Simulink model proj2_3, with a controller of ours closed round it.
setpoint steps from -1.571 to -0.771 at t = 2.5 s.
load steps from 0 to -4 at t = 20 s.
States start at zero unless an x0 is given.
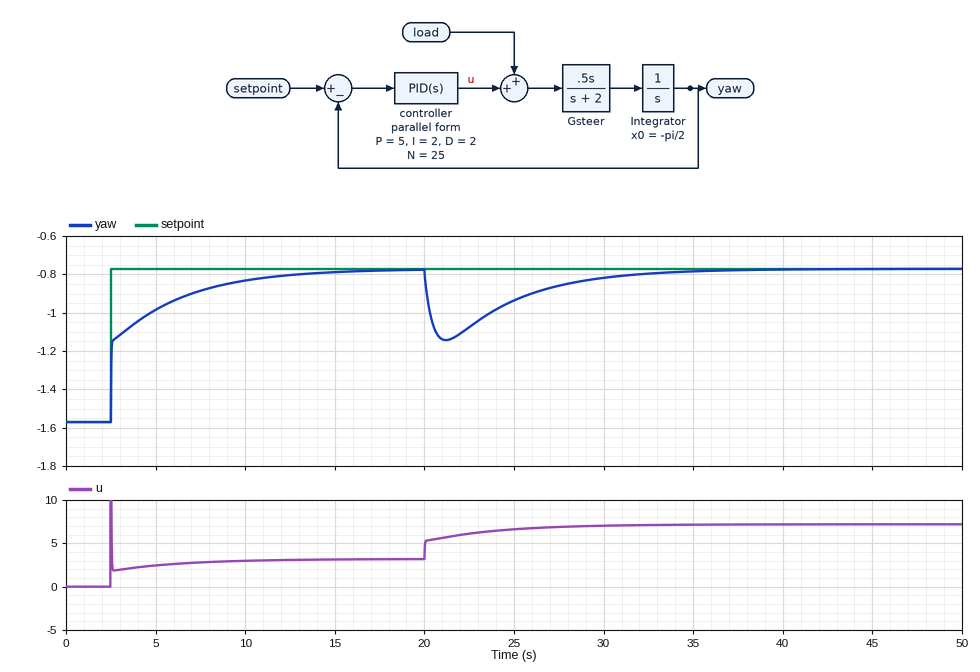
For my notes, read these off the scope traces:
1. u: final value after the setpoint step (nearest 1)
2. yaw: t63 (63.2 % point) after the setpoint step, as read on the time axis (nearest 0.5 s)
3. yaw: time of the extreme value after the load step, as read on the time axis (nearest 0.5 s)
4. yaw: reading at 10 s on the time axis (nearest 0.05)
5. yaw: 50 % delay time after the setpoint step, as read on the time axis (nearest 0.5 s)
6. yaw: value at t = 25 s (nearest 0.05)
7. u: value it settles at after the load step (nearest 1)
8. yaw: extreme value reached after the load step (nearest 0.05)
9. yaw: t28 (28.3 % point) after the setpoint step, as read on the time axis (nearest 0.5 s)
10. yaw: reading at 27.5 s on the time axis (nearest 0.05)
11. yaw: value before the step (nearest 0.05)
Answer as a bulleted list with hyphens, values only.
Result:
- 3
- 3.5 s
- 21.0 s
- -0.85
- 2.5 s
- -0.95
- 7
- -1.15
- 2.5 s
- -0.85
- -1.55
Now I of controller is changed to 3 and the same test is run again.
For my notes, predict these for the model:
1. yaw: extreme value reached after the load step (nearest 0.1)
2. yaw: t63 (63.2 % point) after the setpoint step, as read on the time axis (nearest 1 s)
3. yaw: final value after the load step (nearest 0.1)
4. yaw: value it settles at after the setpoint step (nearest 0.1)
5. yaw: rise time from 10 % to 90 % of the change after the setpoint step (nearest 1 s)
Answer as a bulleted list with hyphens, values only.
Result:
- -1.1
- 3 s
- -0.8
- -0.8
- 4 s
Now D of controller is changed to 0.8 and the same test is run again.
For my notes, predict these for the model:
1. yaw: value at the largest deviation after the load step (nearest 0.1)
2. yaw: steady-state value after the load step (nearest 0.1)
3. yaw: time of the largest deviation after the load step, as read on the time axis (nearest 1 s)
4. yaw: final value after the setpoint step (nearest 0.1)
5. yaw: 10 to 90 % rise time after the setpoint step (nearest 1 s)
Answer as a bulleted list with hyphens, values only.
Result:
- -1.2
- -0.8
- 21 s
- -0.8
- 6 s
